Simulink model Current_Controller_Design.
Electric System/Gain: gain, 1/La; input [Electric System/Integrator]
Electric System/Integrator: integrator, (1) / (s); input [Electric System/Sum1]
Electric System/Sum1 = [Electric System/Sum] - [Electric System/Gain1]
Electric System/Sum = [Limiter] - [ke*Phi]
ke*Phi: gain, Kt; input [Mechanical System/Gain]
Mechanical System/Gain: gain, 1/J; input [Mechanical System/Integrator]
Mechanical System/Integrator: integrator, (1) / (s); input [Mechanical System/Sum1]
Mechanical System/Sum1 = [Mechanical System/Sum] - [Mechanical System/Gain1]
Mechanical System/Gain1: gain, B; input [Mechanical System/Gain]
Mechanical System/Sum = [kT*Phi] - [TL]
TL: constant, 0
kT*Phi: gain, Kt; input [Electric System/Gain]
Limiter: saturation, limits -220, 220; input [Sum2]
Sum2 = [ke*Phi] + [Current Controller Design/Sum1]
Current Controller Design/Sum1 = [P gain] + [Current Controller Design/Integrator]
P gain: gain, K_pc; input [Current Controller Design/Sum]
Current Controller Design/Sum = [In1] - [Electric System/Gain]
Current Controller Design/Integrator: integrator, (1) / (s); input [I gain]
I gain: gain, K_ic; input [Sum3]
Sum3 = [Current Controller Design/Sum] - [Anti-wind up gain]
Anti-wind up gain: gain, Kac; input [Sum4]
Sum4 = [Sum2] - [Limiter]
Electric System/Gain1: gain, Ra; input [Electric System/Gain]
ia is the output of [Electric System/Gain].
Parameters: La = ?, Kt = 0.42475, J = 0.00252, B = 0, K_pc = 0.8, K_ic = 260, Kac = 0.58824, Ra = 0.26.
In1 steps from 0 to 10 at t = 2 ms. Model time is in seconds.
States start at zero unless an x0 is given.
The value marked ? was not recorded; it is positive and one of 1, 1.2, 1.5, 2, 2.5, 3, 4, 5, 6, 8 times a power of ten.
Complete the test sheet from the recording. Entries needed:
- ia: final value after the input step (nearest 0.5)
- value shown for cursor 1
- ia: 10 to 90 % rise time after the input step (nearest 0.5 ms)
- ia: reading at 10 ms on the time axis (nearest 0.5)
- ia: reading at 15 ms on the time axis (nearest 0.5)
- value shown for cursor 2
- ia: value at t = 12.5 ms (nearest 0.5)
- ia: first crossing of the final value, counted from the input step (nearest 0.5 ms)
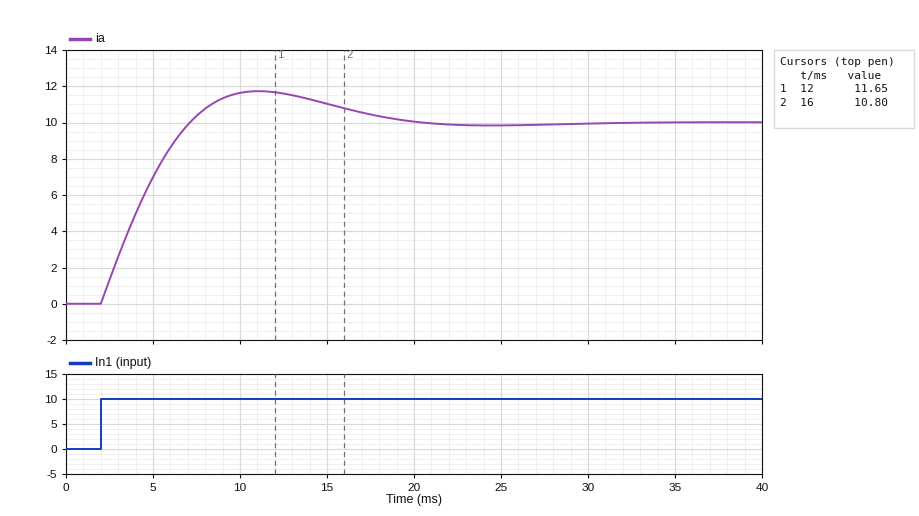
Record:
10.0
11.65
4.0 ms
11.5
11.0
10.80
11.5
5.0 ms
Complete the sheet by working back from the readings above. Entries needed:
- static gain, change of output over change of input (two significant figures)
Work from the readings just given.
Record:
1.0
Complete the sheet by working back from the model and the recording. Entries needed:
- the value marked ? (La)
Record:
0.003
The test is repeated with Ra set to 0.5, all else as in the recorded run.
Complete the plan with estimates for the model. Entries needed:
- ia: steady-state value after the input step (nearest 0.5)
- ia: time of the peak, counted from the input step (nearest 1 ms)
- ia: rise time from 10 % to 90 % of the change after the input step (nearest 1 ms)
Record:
10.0
10 ms
5 ms
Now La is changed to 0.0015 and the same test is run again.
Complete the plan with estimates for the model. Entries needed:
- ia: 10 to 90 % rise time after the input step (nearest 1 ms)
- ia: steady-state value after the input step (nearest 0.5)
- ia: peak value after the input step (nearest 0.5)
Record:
3 ms
10.0
10.5
